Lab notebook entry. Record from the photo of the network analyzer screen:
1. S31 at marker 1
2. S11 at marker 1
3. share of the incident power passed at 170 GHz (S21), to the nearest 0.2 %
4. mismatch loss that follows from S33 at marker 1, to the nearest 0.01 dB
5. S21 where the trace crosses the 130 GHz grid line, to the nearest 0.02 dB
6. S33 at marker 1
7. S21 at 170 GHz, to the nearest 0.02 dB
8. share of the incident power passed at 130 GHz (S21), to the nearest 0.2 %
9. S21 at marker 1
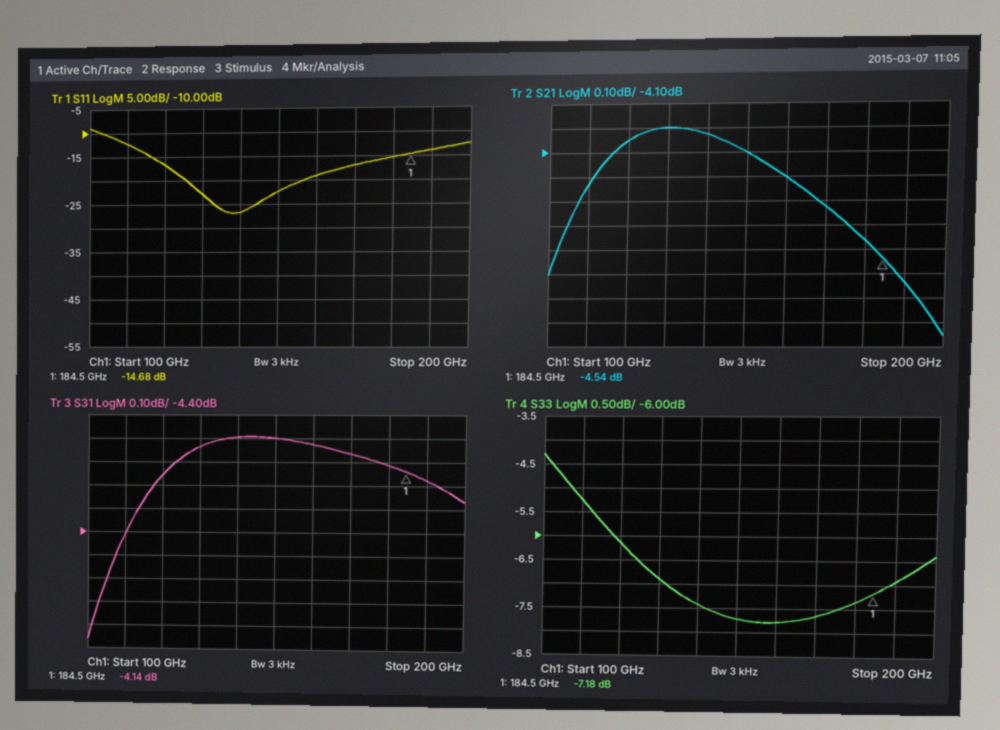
-4.14 dB
-14.68 dB
37.0 %
0.92 dB
-4.00 dB
-7.18 dB
-4.32 dB
39.8 %
-4.54 dB
